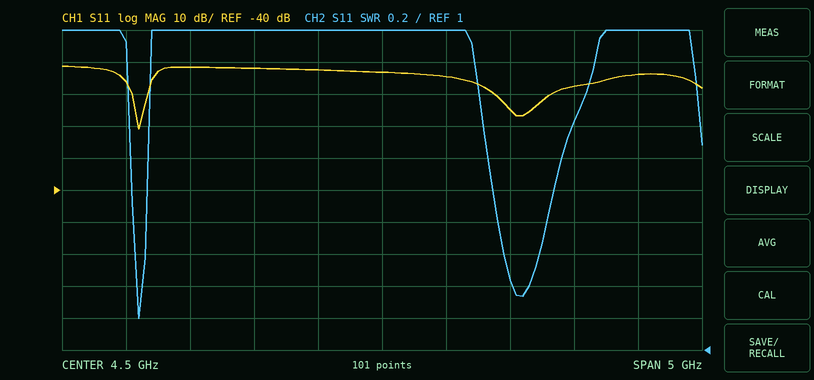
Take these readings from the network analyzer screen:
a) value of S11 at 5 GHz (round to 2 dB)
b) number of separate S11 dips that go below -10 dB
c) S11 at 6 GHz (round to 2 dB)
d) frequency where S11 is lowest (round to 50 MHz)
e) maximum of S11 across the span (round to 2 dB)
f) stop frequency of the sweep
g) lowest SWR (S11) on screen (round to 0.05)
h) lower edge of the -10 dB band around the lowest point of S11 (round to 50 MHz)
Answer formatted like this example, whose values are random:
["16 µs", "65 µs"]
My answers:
["-4 dB", "2", "-8 dB", "2.60 GHz", "-2 dB", "7 GHz", "1.20", "2.55 GHz"]
